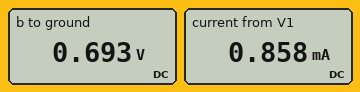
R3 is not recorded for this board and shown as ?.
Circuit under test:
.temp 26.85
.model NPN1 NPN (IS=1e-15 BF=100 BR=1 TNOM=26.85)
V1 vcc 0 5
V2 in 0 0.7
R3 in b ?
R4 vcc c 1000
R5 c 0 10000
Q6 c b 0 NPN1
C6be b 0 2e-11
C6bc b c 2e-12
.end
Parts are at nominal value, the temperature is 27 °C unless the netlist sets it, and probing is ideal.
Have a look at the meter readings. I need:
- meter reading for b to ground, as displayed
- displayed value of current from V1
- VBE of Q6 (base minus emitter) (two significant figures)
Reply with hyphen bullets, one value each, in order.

- 0.693 V
- 0.858 mA
- 690 mV
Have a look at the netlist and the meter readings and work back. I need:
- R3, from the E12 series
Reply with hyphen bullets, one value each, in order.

- 1.5 kΩ
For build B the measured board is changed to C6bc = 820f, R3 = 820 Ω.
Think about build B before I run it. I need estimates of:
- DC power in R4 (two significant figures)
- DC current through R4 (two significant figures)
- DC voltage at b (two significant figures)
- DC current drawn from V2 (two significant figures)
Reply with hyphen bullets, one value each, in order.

- 810 µW
- 900 µA
- 700 mV
- 4.9 µA
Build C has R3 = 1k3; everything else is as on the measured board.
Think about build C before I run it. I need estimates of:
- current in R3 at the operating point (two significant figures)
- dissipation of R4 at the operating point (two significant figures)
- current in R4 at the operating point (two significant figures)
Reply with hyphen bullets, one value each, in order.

- 4.6 µA
- 760 µW
- 870 µA
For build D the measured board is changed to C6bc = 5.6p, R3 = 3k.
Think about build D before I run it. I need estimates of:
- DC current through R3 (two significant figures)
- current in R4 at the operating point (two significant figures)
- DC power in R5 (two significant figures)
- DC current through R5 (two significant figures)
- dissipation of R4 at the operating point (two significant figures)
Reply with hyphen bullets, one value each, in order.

- 3.7 µA
- 790 µA
- 1.8 mW
- 420 µA
- 630 µW
